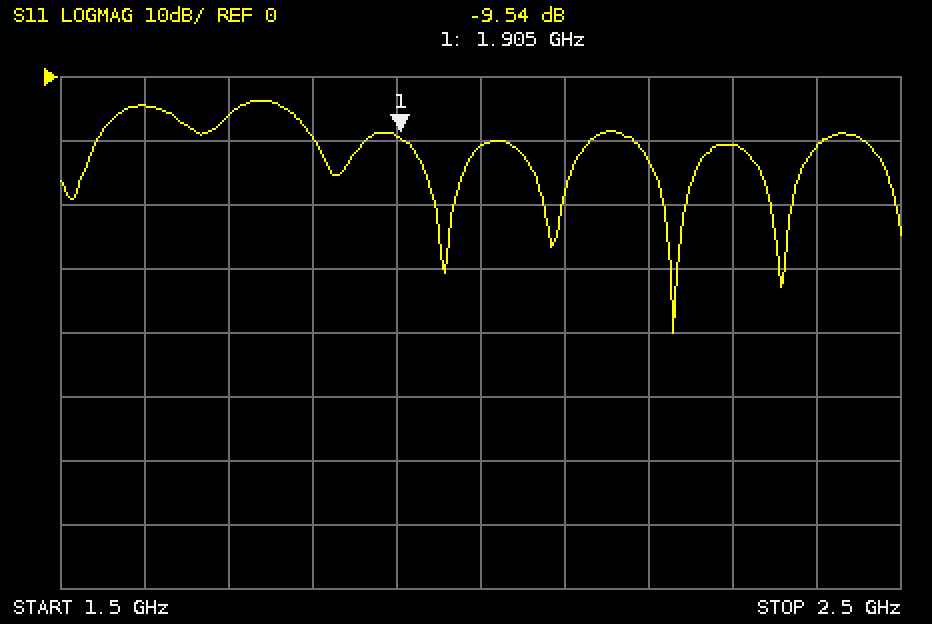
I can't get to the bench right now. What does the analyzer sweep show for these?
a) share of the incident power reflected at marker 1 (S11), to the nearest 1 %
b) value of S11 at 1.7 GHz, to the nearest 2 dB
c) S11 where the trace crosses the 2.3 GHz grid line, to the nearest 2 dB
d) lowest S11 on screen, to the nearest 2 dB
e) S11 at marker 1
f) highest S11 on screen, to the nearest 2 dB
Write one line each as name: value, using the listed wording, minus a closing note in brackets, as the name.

share of the incident power reflected at marker 1 (S11), to the nearest 1 %: 11 %
value of S11 at 1.7 GHz, to the nearest 2 dB: -6 dB
S11 where the trace crosses the 2.3 GHz grid line, to the nearest 2 dB: -10 dB
lowest S11 on screen, to the nearest 2 dB: -40 dB
S11 at marker 1: -9.54 dB
highest S11 on screen, to the nearest 2 dB: -4 dB
